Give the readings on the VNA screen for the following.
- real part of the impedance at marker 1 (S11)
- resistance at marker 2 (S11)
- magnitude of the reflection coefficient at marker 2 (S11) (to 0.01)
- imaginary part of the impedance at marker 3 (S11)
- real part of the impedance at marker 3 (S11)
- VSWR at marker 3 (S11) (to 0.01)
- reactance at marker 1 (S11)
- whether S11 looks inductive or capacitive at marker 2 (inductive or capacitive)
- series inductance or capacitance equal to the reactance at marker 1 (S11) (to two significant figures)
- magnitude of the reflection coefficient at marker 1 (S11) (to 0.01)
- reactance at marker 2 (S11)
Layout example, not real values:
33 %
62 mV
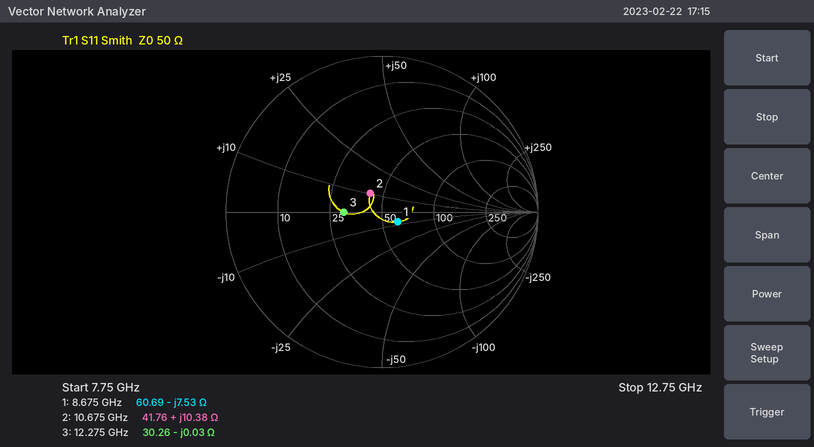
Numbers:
60.69 Ω
41.76 Ω
0.14
-0.03 Ω
30.26 Ω
1.65
-7.53 Ω
inductive
2.4 pF
0.12
+10.38 Ω
